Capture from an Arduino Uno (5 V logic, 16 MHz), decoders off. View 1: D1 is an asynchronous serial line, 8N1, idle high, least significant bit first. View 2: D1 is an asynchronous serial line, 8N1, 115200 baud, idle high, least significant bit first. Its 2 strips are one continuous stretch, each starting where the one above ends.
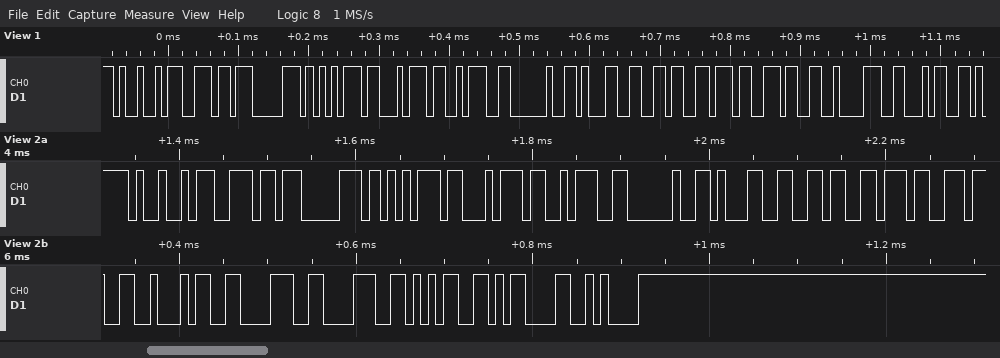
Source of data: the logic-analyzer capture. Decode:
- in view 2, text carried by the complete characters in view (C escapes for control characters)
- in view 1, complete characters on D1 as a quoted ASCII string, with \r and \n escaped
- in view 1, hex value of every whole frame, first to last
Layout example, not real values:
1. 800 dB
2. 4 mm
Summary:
1. "Input: 16734885\r\n"
2. "Input: 167384"
3. 49 6E 70 75 74 3A 20 31 36 37 33 38 34
